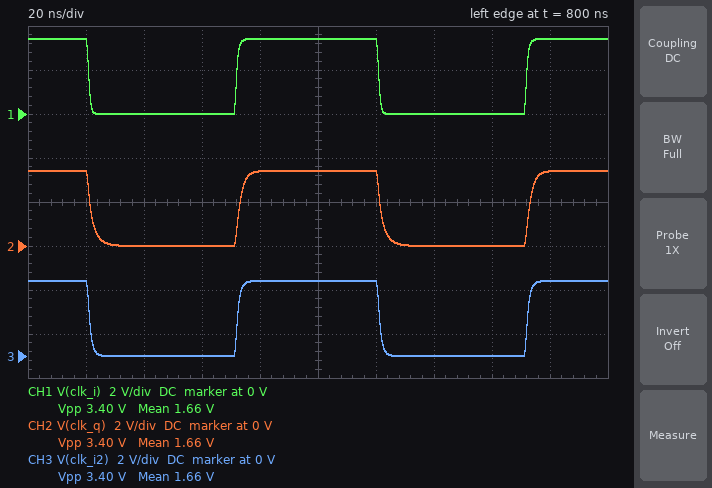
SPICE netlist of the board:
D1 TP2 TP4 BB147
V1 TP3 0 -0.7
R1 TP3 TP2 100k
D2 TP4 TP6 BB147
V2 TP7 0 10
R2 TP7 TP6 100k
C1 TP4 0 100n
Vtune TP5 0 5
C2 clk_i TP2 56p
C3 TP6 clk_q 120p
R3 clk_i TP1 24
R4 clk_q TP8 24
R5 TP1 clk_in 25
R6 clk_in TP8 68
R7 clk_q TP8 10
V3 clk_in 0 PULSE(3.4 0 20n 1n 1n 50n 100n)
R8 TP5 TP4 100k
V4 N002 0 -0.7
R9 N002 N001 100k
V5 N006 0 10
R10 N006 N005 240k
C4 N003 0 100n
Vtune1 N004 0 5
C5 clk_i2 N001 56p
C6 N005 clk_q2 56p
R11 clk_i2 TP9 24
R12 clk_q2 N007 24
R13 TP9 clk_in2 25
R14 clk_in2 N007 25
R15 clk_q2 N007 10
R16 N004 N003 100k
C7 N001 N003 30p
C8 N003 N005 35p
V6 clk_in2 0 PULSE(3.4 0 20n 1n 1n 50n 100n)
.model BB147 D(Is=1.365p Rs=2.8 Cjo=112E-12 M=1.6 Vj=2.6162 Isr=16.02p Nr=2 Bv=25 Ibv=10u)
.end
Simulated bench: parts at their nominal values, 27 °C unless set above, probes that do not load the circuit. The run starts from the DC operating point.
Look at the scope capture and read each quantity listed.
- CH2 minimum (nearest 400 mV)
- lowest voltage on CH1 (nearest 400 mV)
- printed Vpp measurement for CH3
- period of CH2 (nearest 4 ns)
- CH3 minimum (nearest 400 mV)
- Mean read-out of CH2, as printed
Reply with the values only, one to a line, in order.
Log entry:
0 V
0 V
3.40 V
100 ns
0 V
1.66 V
